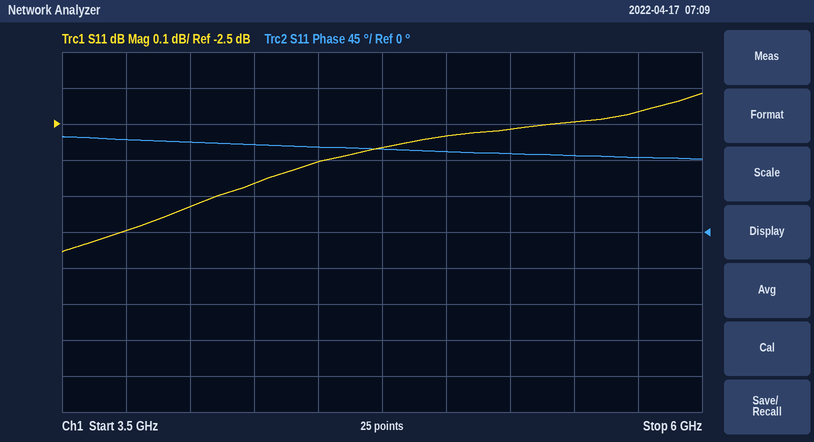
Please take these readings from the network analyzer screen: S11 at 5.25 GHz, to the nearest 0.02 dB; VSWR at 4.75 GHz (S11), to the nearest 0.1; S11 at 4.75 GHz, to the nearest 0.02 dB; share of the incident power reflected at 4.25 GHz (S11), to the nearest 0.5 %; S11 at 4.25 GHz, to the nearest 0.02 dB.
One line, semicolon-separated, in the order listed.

-2.52 dB; 6.8; -2.56 dB; 54.0 %; -2.66 dB
